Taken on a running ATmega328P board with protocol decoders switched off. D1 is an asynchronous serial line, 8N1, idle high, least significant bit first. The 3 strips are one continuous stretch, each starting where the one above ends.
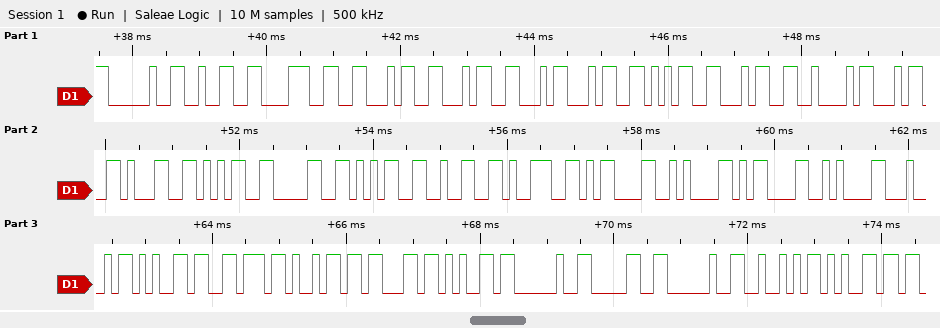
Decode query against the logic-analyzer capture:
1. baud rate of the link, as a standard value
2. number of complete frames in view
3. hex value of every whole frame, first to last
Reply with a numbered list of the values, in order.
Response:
1. 9600 baud
2. 32
3. 0x20 0x32 0x38 0x46 0x46 0x46 0x34 0x35 0x34 0x42 0x34 0x31 0x35 0x30 0x35 0x32 0x39 0x0D 0x0A 0x0D 0x0A 0x44 0x65 0x76 0x69 0x63 0x65 0x20 0x30 0x20 0x52 0x65
